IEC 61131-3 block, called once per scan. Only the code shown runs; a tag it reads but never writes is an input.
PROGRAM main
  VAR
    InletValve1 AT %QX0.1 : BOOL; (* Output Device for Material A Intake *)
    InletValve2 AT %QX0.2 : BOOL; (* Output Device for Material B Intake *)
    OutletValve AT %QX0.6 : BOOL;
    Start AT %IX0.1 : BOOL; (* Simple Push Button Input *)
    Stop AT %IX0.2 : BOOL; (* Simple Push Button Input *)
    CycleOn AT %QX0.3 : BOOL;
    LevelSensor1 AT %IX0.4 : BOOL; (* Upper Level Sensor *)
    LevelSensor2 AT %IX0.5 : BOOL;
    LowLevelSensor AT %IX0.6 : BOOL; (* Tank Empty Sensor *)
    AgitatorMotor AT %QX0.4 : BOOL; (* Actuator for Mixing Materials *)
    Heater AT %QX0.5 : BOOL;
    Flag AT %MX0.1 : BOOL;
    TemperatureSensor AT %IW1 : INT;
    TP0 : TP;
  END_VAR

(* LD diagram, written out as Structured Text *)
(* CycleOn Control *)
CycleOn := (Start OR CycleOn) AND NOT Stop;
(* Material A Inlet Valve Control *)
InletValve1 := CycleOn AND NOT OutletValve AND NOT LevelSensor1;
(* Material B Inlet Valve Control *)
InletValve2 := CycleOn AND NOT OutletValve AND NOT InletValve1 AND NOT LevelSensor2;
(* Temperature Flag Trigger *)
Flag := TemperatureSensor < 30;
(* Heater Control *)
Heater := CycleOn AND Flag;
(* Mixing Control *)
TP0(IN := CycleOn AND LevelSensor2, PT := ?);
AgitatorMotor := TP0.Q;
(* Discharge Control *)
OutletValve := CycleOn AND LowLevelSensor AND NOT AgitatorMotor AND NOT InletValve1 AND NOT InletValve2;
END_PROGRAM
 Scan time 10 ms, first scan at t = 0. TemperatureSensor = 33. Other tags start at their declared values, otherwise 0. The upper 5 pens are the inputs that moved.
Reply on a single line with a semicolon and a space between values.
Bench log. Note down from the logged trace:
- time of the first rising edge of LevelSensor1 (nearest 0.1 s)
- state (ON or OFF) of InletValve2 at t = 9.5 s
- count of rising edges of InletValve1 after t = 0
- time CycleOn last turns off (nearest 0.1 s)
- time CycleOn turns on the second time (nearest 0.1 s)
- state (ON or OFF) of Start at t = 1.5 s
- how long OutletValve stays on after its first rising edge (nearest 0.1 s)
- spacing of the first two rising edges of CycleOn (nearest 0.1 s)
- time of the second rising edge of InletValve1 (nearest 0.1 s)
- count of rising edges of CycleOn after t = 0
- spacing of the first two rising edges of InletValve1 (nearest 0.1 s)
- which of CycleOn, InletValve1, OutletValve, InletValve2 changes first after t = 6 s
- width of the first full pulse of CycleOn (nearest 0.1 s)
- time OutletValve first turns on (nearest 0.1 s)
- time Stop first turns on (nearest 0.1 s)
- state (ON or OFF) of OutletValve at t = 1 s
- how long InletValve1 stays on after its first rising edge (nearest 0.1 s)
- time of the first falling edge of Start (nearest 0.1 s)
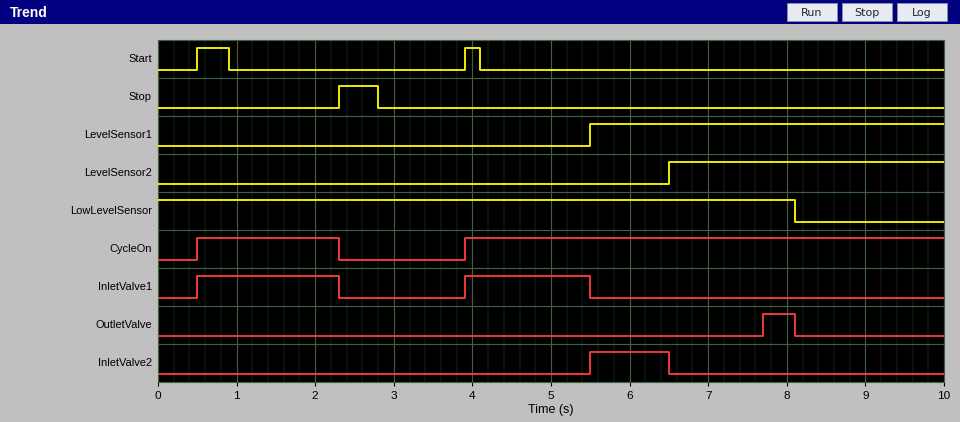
5.5 s; OFF; 2; 2.3 s; 3.9 s; OFF; 0.4 s; 3.4 s; 3.9 s; 2; 3.4 s; InletValve2; 1.8 s; 7.7 s; 2.3 s; OFF; 1.8 s; 0.9 s
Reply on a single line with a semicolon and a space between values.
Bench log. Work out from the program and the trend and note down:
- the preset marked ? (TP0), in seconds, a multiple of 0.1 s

1.2 s
